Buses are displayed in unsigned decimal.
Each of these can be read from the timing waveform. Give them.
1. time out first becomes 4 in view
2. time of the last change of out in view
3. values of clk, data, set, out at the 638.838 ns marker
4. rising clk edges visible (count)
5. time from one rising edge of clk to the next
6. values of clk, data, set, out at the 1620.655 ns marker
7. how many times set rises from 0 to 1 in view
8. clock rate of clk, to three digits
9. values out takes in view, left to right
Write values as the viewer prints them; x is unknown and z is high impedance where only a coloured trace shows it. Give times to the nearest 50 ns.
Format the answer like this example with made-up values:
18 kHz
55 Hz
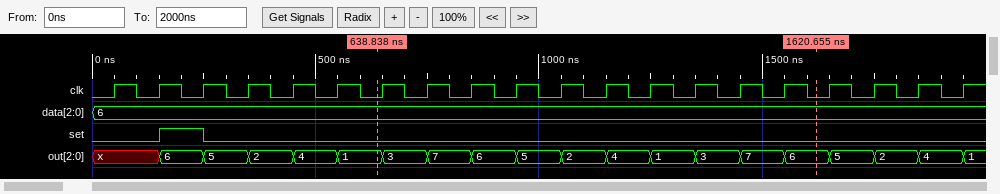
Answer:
450 ns
1950 ns
clk=0, data=6, set=0, out=1
20
100 ns
clk=0, data=6, set=0, out=6
1
10.0 MHz
x, 6, 5, 2, 4, 1, 3, 7, 6, 5, 2, 4, 1, 3, 7, 6, 5, 2, 4, 1
